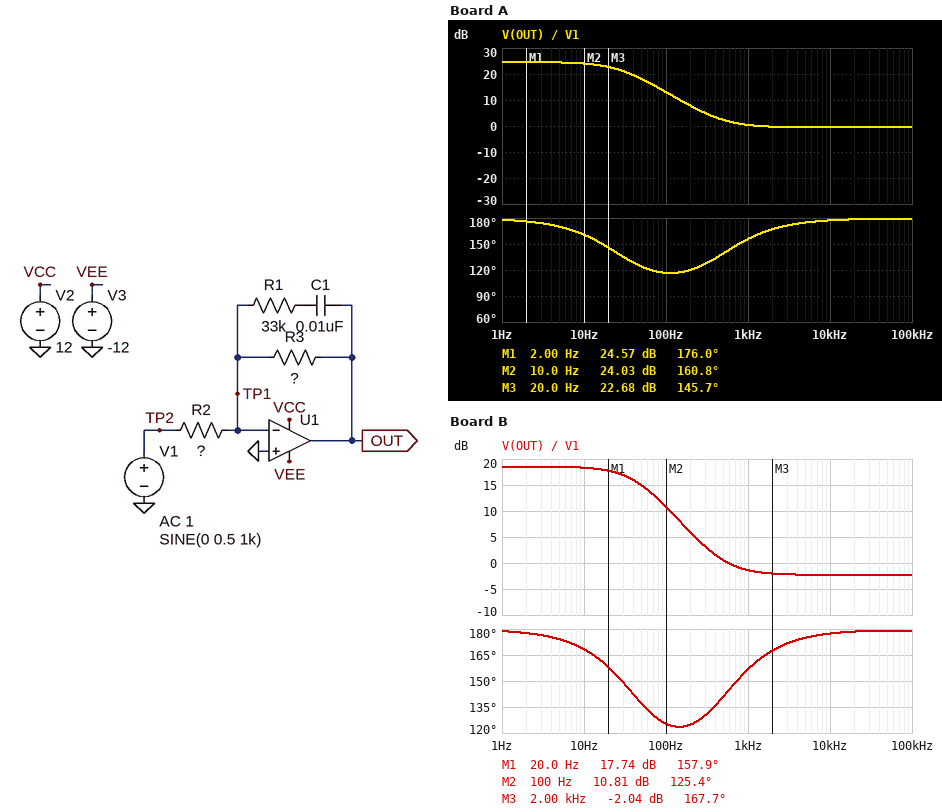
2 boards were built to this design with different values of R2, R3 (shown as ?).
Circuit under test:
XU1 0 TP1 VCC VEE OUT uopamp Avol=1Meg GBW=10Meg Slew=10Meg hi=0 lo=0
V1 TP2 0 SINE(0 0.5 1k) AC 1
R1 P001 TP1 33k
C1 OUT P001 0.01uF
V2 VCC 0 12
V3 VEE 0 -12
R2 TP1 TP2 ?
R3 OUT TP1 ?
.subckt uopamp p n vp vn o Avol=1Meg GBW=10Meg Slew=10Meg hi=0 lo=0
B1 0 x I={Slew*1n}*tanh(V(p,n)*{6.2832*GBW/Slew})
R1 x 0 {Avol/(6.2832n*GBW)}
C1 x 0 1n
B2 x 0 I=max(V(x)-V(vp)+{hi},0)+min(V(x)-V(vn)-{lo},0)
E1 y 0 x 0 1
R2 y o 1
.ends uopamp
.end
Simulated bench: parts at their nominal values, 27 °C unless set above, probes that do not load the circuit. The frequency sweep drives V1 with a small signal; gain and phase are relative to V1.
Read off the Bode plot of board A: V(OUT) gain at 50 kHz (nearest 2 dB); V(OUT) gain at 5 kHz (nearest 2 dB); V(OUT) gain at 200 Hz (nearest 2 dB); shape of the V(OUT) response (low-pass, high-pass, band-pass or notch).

0 dB
0 dB
8 dB
low-pass
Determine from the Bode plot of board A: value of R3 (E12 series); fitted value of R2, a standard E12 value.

560 kΩ
33 kΩ
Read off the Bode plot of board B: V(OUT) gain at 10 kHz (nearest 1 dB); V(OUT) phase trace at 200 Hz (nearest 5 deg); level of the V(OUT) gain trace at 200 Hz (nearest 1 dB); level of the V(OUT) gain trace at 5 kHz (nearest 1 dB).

-2 dB
125 deg
6 dB
-2 dB
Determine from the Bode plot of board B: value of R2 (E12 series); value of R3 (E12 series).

39 kΩ
330 kΩ
